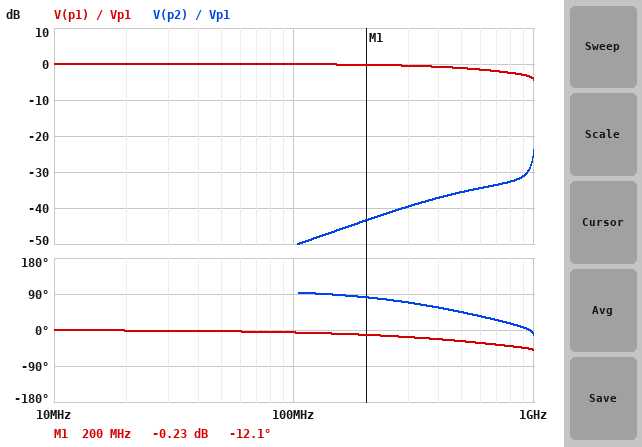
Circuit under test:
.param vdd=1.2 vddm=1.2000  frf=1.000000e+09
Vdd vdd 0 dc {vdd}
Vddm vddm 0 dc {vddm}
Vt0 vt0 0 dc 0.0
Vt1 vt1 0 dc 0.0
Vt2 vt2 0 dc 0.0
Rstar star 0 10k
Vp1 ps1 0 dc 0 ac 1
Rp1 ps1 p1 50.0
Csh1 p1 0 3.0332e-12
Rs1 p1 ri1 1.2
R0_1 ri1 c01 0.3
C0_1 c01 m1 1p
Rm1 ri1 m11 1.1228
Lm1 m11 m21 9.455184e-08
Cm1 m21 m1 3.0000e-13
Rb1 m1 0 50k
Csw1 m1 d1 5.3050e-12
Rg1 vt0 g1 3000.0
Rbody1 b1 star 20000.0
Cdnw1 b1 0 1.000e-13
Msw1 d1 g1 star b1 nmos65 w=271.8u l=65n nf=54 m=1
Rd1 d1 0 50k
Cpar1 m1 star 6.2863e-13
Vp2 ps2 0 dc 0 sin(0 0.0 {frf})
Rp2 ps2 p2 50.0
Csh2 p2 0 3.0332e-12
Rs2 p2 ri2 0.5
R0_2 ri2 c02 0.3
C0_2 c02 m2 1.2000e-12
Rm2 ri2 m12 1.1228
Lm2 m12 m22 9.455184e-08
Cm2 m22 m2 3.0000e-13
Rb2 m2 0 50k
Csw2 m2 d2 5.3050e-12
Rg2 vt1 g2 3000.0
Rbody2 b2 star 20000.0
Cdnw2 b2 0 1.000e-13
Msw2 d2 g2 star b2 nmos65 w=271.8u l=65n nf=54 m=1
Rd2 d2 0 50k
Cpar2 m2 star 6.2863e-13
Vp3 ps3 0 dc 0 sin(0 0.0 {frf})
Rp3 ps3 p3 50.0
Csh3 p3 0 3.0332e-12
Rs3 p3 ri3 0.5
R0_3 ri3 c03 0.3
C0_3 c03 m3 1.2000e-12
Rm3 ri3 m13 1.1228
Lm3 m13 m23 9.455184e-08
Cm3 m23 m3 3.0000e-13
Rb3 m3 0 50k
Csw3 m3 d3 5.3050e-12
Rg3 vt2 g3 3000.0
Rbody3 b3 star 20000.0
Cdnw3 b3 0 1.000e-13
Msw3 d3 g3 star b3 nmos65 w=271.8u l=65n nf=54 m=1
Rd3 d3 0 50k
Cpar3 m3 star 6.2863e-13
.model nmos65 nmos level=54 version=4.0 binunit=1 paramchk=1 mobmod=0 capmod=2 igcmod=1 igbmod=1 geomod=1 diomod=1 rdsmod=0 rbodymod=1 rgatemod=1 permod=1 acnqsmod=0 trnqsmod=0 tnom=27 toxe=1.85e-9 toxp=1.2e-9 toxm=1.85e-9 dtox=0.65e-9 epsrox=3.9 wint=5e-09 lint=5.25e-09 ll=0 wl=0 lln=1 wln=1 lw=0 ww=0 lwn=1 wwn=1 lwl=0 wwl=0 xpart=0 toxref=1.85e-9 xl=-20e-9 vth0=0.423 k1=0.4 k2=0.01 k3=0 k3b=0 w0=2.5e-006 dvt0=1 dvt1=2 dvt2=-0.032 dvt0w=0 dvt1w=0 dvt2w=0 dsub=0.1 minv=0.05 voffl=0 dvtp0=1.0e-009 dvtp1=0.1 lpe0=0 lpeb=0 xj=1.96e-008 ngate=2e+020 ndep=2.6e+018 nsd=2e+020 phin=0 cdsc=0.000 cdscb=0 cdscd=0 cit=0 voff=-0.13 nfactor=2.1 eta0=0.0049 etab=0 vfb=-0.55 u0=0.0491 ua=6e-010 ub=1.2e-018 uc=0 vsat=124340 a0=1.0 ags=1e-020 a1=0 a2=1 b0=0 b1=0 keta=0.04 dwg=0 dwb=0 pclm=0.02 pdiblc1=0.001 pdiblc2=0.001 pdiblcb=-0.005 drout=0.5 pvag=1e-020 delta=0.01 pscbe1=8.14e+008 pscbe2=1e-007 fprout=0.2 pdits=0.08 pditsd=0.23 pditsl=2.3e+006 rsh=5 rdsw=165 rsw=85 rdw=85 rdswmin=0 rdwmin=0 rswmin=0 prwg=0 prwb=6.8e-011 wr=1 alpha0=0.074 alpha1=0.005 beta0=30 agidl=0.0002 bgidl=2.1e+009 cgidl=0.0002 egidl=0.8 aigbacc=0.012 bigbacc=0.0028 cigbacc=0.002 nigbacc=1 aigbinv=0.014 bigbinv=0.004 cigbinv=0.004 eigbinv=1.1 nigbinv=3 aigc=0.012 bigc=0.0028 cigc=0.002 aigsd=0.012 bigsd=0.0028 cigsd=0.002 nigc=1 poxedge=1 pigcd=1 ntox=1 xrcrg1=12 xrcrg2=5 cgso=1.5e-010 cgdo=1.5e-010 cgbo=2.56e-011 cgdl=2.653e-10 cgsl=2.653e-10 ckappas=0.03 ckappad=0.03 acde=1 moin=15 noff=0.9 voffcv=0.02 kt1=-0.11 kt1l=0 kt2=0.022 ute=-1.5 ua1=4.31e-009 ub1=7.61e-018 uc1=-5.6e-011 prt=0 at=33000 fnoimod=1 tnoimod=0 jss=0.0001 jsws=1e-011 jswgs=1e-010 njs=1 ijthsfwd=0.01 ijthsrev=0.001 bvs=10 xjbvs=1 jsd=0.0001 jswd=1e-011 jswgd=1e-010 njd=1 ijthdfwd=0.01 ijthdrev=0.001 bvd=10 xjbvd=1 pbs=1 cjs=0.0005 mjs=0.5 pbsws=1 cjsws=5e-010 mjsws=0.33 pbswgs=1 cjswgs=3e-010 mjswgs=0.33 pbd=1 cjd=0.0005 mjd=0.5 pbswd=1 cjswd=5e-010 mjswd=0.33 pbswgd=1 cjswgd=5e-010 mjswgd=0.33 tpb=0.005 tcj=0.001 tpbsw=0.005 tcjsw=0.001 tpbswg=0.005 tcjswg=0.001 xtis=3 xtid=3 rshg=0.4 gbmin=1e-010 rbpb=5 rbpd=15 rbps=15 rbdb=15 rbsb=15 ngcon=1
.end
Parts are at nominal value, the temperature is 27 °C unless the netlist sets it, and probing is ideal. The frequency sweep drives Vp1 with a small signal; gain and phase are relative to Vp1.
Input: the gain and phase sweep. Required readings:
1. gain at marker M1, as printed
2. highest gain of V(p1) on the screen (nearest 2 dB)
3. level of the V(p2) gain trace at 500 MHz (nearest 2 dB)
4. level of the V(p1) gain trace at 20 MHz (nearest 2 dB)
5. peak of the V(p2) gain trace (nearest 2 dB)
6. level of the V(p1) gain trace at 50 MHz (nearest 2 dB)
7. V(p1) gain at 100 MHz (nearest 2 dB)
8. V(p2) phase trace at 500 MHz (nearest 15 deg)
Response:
-0.23 dB
0 dB
-36 dB
0 dB
-24 dB
0 dB
0 dB
45 deg
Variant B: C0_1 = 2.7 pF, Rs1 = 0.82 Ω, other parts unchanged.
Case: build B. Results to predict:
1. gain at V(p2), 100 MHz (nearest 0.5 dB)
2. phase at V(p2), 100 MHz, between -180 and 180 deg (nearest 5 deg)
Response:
-48.5 dB
90 deg
